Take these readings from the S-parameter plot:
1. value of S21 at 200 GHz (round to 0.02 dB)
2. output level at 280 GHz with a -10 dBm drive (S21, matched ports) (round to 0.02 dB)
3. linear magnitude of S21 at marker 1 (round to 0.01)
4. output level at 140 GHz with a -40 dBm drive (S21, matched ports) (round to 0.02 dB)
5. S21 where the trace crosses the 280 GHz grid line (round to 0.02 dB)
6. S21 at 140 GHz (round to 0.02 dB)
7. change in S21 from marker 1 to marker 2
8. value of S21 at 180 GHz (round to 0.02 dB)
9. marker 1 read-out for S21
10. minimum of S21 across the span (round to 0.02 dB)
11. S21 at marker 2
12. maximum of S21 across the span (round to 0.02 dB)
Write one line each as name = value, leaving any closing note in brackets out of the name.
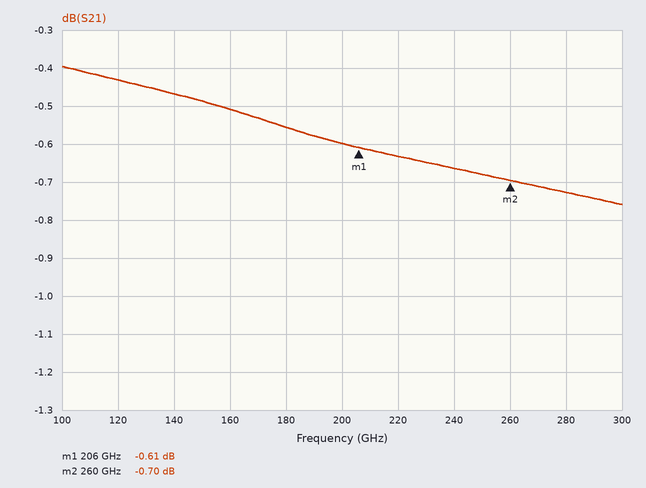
value of S21 at 200 GHz = -0.60 dB
output level at 280 GHz with a -10 dBm drive (S21, matched ports) = -10.72 dBm
linear magnitude of S21 at marker 1 = 0.93
output level at 140 GHz with a -40 dBm drive (S21, matched ports) = -40.46 dBm
S21 where the trace crosses the 280 GHz grid line = -0.72 dB
S21 at 140 GHz = -0.46 dB
change in S21 from marker 1 to marker 2 = -0.09 dB
value of S21 at 180 GHz = -0.56 dB
marker 1 read-out for S21 = -0.61 dB
minimum of S21 across the span = -0.76 dB
S21 at marker 2 = -0.70 dB
maximum of S21 across the span = -0.40 dB
